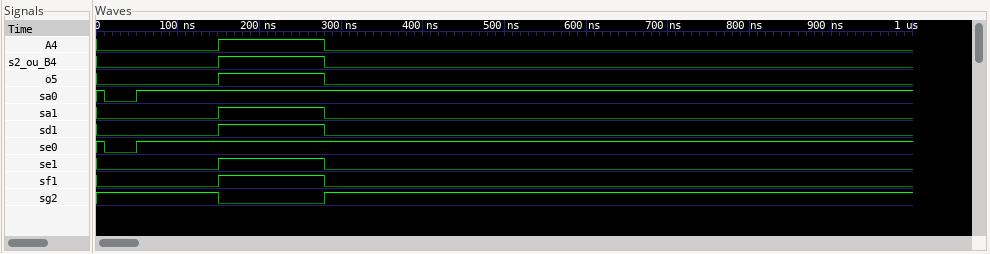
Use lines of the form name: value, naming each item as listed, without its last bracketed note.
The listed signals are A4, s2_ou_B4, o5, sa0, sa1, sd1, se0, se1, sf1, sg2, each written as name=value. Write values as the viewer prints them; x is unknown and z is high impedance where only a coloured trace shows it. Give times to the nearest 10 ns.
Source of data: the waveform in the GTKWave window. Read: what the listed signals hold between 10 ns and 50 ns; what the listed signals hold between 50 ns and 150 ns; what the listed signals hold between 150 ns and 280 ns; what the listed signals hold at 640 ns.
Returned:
what the listed signals hold between 10 ns and 50 ns: A4=0, s2_ou_B4=0, o5=0, sa0=0, sa1=0, sd1=0, se0=0, se1=0, sf1=0, sg2=1
what the listed signals hold between 50 ns and 150 ns: A4=0, s2_ou_B4=0, o5=0, sa0=1, sa1=0, sd1=0, se0=1, se1=0, sf1=0, sg2=1
what the listed signals hold between 150 ns and 280 ns: A4=1, s2_ou_B4=1, o5=1, sa0=1, sa1=1, sd1=1, se0=1, se1=1, sf1=1, sg2=0
what the listed signals hold at 640 ns: A4=0, s2_ou_B4=0, o5=0, sa0=1, sa1=0, sd1=0, se0=1, se1=0, sf1=0, sg2=1
